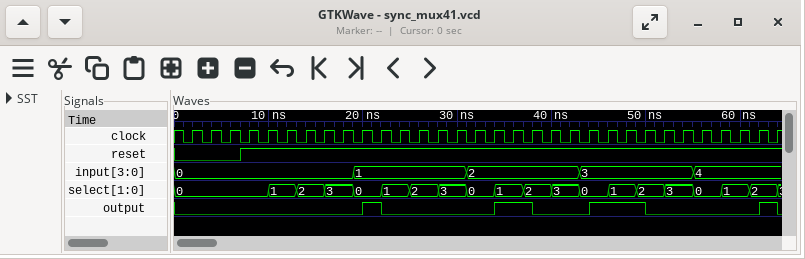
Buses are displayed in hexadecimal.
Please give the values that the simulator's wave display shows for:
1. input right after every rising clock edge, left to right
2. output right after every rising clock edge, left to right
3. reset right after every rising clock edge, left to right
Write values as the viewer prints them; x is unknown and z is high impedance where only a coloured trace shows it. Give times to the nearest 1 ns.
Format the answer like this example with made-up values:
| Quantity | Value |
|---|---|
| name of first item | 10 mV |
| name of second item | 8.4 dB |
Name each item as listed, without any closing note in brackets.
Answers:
| Quantity | Value |
|---|---|
| input right after every rising clock edge, left to right | 0, 0, 0, 0, 0, 0, 0, 0, 0, 1, 1, 1, 1, 1, 1, 2, 2, 2, 2, 2, 2, 3, 3, 3, 3, 3, 3, 4, 4, 4, 4, 4 |
| output right after every rising clock edge, left to right | 0 0 0 0 0 0 0 0 0 1 0 0 0 0 0 0 1 1 0 0 0 1 1 1 0 0 0 0 0 0 1 0 |
| reset right after every rising clock edge, left to right | 0 0 0 1 1 1 1 1 1 1 1 1 1 1 1 1 1 1 1 1 1 1 1 1 1 1 1 1 1 1 1 1 |
